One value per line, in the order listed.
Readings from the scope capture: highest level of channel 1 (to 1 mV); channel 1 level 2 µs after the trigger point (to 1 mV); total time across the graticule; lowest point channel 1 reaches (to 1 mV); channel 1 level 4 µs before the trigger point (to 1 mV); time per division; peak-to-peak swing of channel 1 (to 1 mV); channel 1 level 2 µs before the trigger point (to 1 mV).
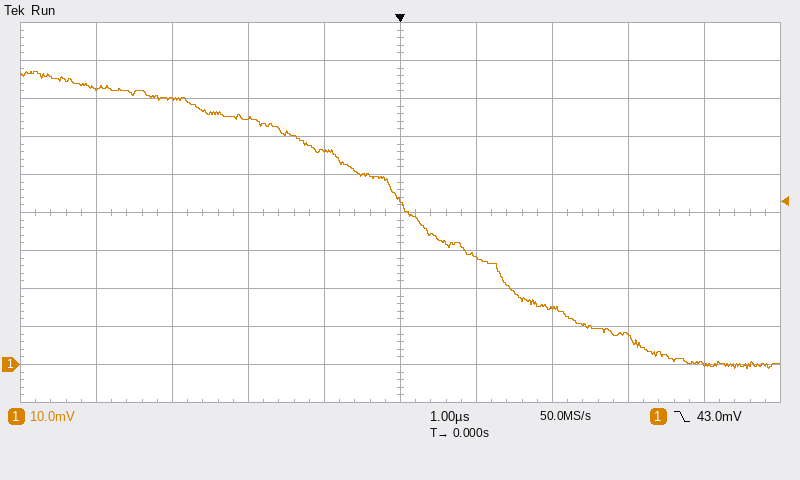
77 mV
15 mV
10 µs
-1 mV
73 mV
1 µs
78 mV
65 mV
